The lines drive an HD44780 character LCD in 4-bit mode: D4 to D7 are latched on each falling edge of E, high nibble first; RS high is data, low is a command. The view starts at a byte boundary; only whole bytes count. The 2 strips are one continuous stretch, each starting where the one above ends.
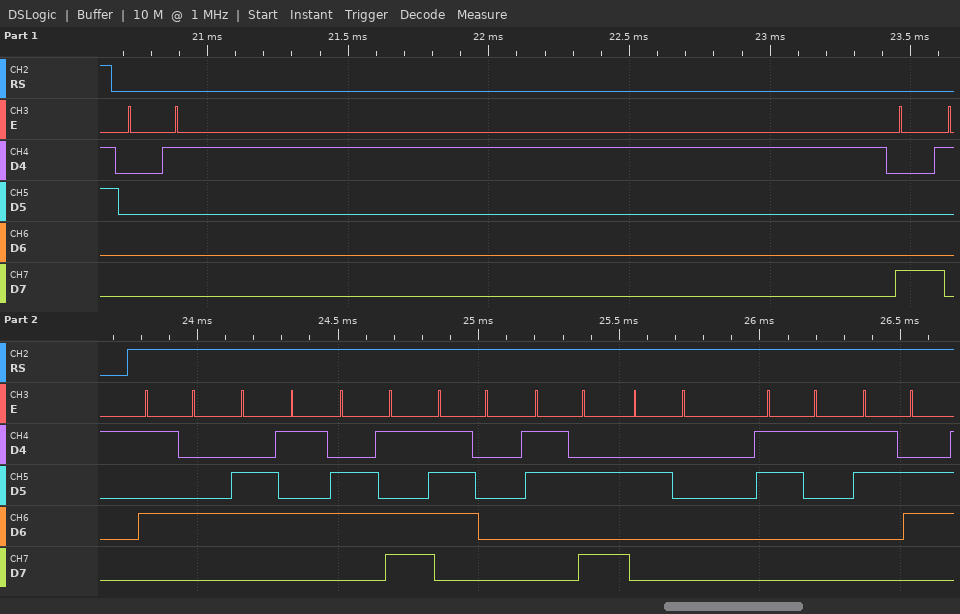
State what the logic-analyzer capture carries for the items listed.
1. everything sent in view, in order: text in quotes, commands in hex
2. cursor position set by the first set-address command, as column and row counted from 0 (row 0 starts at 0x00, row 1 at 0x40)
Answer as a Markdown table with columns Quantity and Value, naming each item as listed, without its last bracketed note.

| Quantity | Value |
|---|---|
| everything sent in view, in order: text in quotes, commands in hex | 0x01 0x81 "Temp: 16" |
| cursor position set by the first set-address command, as column and row counted from 0 | column 1, row 0 |
